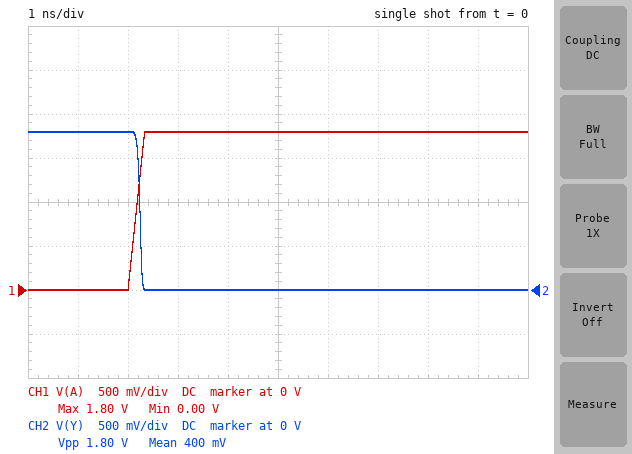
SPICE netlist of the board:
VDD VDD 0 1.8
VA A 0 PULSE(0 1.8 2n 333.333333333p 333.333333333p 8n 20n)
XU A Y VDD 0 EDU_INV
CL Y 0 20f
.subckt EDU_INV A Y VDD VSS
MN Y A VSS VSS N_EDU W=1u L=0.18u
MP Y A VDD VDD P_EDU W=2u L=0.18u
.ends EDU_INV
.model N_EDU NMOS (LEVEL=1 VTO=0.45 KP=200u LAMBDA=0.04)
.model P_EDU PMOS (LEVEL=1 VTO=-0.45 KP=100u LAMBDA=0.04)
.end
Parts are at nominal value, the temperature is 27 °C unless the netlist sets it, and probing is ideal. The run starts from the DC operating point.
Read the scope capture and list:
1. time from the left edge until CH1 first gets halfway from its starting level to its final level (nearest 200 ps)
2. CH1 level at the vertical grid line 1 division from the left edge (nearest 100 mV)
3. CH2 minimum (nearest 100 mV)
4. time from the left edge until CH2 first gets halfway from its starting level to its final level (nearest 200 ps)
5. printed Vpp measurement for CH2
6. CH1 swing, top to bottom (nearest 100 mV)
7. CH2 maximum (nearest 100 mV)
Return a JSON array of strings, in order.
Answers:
["2.2 ns", "0 V", "0 V", "2.2 ns", "1.80 V", "1.8 V", "1.8 V"]
